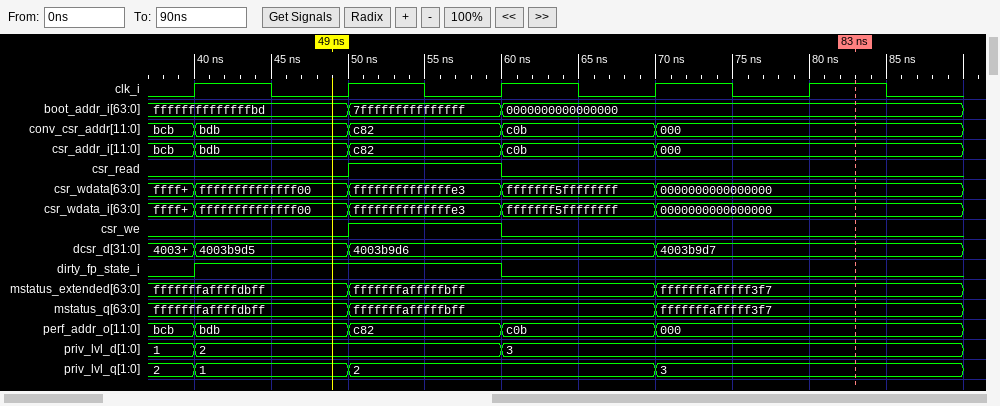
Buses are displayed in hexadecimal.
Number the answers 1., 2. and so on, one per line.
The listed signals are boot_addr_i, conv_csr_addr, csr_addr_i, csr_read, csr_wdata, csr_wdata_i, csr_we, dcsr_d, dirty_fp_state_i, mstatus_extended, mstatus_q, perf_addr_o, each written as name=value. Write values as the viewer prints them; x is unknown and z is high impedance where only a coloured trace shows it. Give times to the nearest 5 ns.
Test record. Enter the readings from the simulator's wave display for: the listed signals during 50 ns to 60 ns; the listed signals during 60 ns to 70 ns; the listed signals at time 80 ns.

1. boot_addr_i=7fffffffffffffff, conv_csr_addr=c82, csr_addr_i=c82, csr_read=1, csr_wdata=ffffffffffffffe3, csr_wdata_i=ffffffffffffffe3, csr_we=1, dcsr_d=4003b9d6, dirty_fp_state_i=1, mstatus_extended=fffffffafffffbff, mstatus_q=fffffffafffffbff, perf_addr_o=c82
2. boot_addr_i=0000000000000000, conv_csr_addr=c0b, csr_addr_i=c0b, csr_read=0, csr_wdata=fffffff5ffffffff, csr_wdata_i=fffffff5ffffffff, csr_we=0, dcsr_d=4003b9d6, dirty_fp_state_i=0, mstatus_extended=fffffffafffffbff, mstatus_q=fffffffafffffbff, perf_addr_o=c0b
3. boot_addr_i=0000000000000000, conv_csr_addr=000, csr_addr_i=000, csr_read=0, csr_wdata=0000000000000000, csr_wdata_i=0000000000000000, csr_we=0, dcsr_d=4003b9d7, dirty_fp_state_i=0, mstatus_extended=fffffffafffff3f7, mstatus_q=fffffffafffff3f7, perf_addr_o=000
